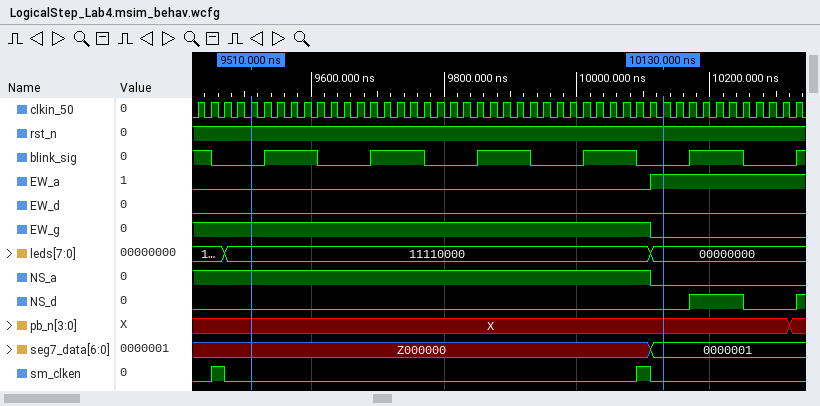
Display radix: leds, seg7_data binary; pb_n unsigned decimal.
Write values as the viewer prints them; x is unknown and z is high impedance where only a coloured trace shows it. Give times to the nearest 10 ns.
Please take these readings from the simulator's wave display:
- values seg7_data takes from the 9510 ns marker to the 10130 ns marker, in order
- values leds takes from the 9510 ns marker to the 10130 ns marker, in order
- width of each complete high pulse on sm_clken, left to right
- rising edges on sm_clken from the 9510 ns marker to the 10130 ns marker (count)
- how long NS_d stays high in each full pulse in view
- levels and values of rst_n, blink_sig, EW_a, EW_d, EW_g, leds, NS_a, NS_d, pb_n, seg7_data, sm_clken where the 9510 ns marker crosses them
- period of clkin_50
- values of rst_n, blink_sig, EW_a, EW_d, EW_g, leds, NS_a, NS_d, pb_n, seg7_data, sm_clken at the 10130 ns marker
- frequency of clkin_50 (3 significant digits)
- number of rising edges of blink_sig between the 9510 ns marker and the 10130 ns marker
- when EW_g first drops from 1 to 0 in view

Z000000, 0000001
11110000, 00000000
20 ns, 20 ns
1
80 ns
rst_n=1, blink_sig=0, EW_a=0, EW_d=0, EW_g=1, leds=11110000, NS_a=1, NS_d=0, pb_n=X, seg7_data=Z000000, sm_clken=0
20 ns
rst_n=1, blink_sig=0, EW_a=1, EW_d=0, EW_g=0, leds=00000000, NS_a=0, NS_d=0, pb_n=X, seg7_data=0000001, sm_clken=0
50.0 MHz
4
10110 ns
